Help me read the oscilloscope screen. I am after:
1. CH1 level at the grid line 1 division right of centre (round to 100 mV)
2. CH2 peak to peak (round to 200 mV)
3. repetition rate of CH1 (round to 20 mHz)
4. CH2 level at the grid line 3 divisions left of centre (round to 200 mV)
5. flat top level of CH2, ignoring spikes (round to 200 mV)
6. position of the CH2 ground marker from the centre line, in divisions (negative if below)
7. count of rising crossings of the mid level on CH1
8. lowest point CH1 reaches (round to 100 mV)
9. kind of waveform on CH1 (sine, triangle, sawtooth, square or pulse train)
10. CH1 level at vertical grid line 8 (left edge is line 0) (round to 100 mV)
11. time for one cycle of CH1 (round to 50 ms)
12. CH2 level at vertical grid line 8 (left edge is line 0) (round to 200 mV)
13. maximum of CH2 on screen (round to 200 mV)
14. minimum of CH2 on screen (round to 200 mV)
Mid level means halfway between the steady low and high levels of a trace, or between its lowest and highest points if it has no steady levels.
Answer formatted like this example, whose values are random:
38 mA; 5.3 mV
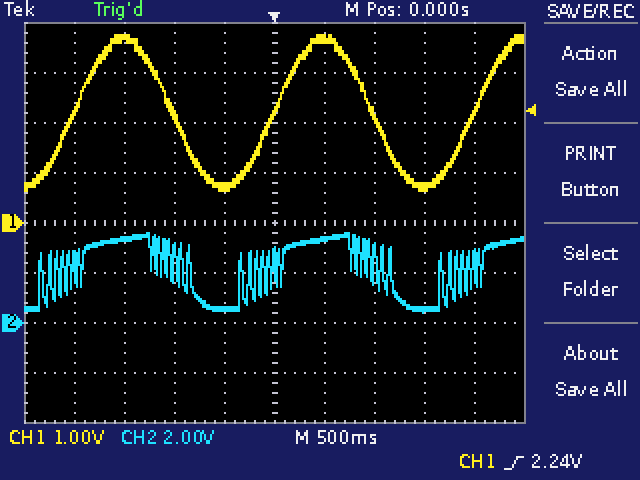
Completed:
3.7 V; 3.2 V; 500 mHz; 3.4 V; 3.2 V; -2.0 div; 3; 600 mV; sine; 700 mV; 2.00 s; 600 mV; 3.6 V; 400 mV
